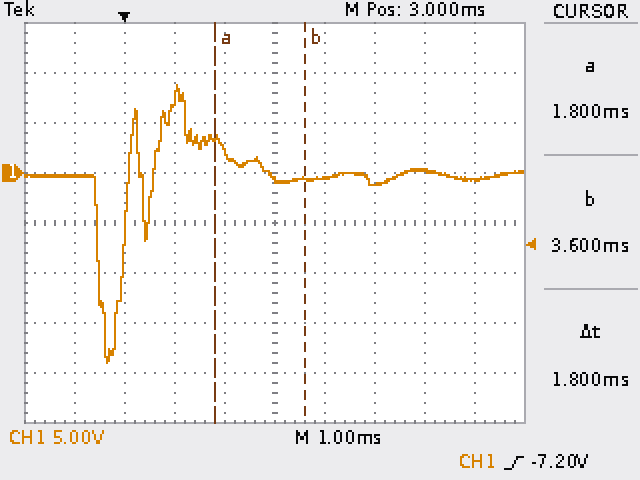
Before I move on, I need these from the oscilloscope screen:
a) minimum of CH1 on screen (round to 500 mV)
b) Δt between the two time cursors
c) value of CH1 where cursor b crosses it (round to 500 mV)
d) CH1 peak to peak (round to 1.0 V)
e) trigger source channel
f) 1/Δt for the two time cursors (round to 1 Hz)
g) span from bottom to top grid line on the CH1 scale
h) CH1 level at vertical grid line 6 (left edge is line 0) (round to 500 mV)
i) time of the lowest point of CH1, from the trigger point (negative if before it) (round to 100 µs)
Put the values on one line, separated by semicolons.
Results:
-19.0 V; 1.8 ms; -500 mV; 28.0 V; CH1; 556 Hz; 40 V; -500 mV; -300 µs
